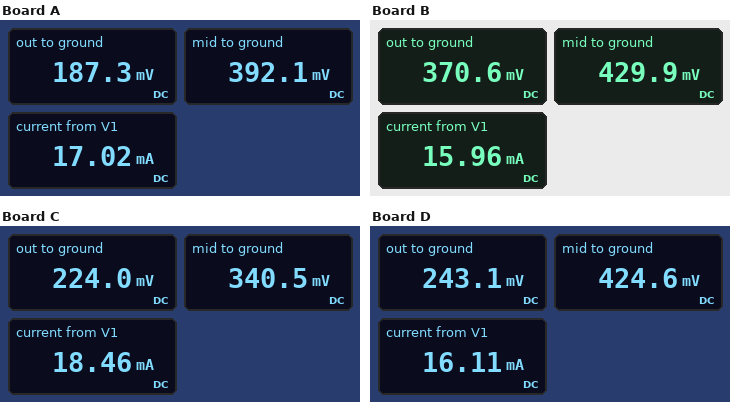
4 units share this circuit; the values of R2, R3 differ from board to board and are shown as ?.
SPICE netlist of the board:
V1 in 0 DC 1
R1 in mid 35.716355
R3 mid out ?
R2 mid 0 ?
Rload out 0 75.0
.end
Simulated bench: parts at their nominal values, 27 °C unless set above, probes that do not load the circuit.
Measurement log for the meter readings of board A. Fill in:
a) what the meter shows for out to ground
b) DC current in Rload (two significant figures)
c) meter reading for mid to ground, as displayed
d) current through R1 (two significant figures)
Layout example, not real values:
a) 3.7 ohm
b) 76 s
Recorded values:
a) 187.3 mV
b) 2.5 mA
c) 392.1 mV
d) 17 mA
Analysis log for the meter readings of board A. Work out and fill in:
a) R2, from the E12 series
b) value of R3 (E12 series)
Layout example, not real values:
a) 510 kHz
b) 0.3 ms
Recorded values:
a) 27 Ω
b) 82 Ω
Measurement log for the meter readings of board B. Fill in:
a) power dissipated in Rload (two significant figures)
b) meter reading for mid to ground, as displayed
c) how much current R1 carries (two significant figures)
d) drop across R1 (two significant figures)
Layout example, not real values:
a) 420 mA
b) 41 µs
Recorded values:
a) 1.8 mW
b) 429.9 mV
c) 16 mA
d) 570 mV
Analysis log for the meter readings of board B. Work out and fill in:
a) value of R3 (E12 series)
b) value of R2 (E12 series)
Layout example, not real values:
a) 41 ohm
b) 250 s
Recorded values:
a) 12 Ω
b) 39 Ω
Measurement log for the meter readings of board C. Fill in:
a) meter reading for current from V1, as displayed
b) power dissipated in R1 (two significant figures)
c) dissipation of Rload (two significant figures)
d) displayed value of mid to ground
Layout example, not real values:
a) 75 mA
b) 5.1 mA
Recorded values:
a) 18.46 mA
b) 12 mW
c) 670 µW
d) 340.5 mV
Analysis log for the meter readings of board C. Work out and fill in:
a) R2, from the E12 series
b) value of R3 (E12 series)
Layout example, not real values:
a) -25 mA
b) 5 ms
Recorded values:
a) 22 Ω
b) 39 Ω
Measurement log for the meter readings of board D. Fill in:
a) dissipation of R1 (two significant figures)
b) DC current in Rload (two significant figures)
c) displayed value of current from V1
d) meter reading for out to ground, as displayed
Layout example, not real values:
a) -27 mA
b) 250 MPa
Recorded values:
a) 9.3 mW
b) 3.2 mA
c) 16.11 mA
d) 243.1 mV
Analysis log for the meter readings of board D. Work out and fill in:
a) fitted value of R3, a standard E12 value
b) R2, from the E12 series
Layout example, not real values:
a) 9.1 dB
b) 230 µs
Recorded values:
a) 56 Ω
b) 33 Ω
